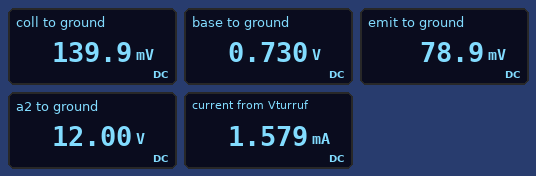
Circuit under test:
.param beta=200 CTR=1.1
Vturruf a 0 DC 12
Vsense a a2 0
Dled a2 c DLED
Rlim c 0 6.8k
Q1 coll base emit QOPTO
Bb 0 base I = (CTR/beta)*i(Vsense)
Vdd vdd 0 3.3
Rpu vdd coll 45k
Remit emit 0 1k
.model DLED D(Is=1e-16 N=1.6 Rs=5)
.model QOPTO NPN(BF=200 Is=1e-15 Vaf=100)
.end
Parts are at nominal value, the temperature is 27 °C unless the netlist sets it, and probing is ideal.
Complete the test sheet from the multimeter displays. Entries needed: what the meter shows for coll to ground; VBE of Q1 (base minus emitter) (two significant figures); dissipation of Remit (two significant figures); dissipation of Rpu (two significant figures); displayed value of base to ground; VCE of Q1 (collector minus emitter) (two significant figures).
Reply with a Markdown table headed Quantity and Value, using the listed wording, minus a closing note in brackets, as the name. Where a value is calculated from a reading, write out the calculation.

| Quantity | Value |
|---|---|
| what the meter shows for coll to ground | 139.9 mV |
| VBE of Q1 (base minus emitter) | 730 mV - 78.9 mV = 650 mV |
| dissipation of Remit | (78.9 mV)^2 / 1 kΩ = 6.2 µW |
| dissipation of Rpu | (3.3 V - 139.9 mV)^2 / 45 kΩ = 220 µW |
| displayed value of base to ground | 0.730 V |
| VCE of Q1 (collector minus emitter) | 139.9 mV - 78.9 mV = 61 mV |
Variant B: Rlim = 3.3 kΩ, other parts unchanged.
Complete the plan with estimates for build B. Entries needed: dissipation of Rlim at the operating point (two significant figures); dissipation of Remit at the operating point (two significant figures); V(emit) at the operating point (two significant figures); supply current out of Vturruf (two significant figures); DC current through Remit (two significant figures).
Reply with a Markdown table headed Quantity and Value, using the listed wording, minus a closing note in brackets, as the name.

| Quantity | Value |
|---|---|
| dissipation of Rlim at the operating point | 35 mW |
| dissipation of Remit at the operating point | 7.8 µW |
| V(emit) at the operating point | 88 mV |
| supply current out of Vturruf | 3.2 mA |
| DC current through Remit | 88 µA |
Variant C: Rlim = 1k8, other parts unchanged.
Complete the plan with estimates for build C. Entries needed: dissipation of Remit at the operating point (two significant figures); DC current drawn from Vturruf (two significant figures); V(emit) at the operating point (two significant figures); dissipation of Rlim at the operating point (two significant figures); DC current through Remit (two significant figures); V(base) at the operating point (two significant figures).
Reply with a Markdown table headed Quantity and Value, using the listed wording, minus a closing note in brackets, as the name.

| Quantity | Value |
|---|---|
| dissipation of Remit at the operating point | 11 µW |
| DC current drawn from Vturruf | 5.9 mA |
| V(emit) at the operating point | 100 mV |
| dissipation of Rlim at the operating point | 63 mW |
| DC current through Remit | 100 µA |
| V(base) at the operating point | 770 mV |
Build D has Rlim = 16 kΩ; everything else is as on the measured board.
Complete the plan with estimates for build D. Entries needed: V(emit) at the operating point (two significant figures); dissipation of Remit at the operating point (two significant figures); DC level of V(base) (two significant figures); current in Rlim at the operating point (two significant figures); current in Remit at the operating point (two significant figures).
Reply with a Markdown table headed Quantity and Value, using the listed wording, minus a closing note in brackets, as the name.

| Quantity | Value |
|---|---|
| V(emit) at the operating point | 74 mV |
| dissipation of Remit at the operating point | 5.4 µW |
| DC level of V(base) | 720 mV |
| current in Rlim at the operating point | 670 µA |
| current in Remit at the operating point | 74 µA |
